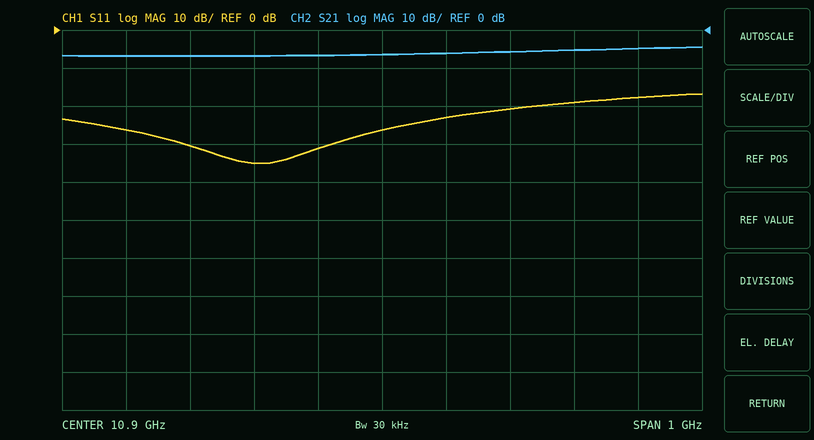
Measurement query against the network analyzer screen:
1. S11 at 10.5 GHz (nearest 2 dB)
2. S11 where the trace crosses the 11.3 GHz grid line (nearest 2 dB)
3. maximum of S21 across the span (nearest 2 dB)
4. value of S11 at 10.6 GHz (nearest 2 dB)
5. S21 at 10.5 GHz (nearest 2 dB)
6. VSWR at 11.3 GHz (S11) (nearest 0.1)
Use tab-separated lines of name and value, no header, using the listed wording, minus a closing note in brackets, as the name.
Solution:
S11 at 10.5 GHz	-26 dB
S11 where the trace crosses the 11.3 GHz grid line	-18 dB
maximum of S21 across the span	-4 dB
value of S11 at 10.6 GHz	-30 dB
S21 at 10.5 GHz	-6 dB
VSWR at 11.3 GHz (S11)	1.3
